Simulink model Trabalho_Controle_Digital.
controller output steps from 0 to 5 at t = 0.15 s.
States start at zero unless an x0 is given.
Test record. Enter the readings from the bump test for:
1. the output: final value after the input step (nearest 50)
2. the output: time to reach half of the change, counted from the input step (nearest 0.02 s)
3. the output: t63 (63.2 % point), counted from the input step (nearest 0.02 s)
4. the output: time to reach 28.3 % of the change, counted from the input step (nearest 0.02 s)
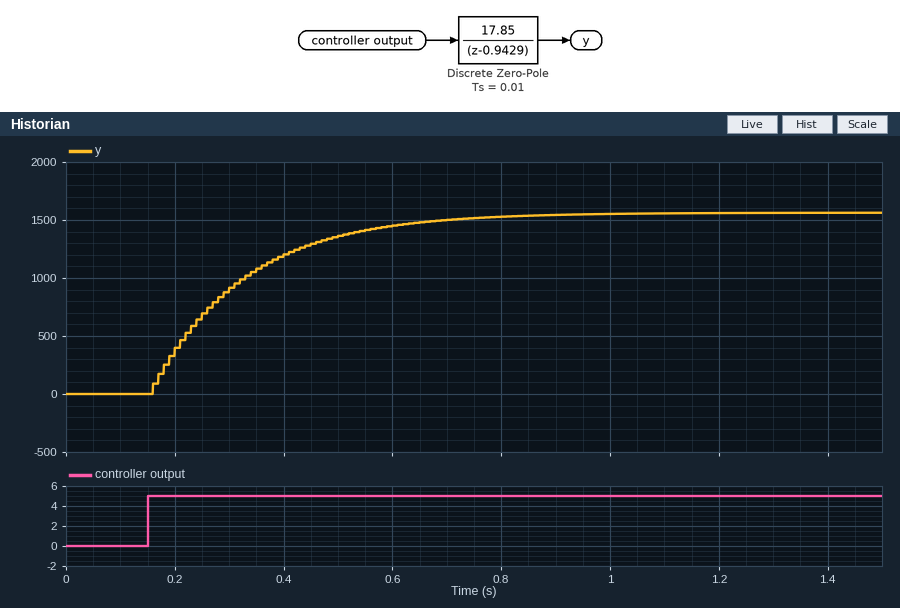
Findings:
1550
0.12 s
0.18 s
0.06 s
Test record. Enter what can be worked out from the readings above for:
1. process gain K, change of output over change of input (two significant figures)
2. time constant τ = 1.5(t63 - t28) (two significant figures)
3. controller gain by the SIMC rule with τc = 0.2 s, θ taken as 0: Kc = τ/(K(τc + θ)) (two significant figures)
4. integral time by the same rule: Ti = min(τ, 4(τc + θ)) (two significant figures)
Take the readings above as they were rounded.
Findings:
310
0.18 s
0.0029
0.18 s
